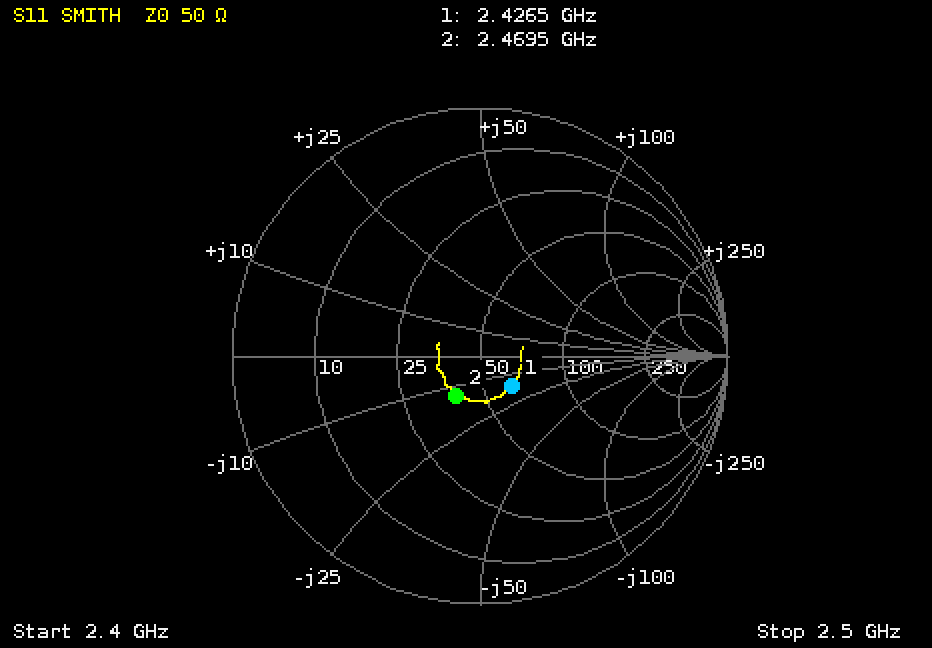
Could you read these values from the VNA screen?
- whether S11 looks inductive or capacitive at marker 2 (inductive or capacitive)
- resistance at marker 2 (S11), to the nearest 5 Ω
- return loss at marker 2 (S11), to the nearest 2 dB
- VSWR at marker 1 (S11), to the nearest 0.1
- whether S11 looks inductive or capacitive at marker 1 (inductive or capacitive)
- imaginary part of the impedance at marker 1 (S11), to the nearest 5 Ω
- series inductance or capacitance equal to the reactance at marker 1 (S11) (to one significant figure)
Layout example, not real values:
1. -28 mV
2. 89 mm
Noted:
1. capacitive
2. 40 Ω
3. 14 dB
4. 1.4
5. capacitive
6. -15 Ω
7. 4 pF
